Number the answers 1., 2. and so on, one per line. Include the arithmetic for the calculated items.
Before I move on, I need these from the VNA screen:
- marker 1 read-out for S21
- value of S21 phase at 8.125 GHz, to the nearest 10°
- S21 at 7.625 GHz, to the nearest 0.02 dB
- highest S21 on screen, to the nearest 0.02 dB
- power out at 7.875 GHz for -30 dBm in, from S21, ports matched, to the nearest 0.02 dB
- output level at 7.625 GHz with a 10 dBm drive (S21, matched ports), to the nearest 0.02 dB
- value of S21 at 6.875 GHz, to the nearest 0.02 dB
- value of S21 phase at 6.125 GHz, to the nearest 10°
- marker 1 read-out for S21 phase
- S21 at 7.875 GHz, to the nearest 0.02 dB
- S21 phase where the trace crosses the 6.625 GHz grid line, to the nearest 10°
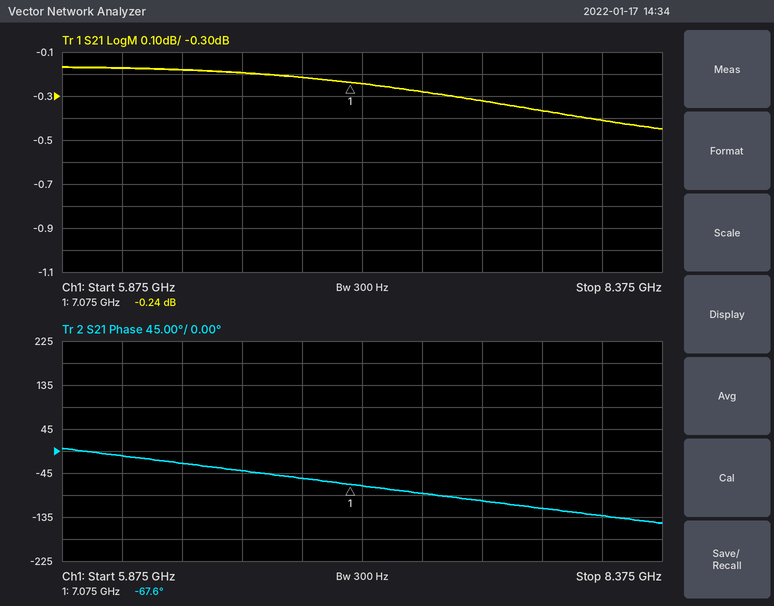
1. -0.24 dB
2. -130°
3. -0.32 dB
4. -0.16 dB
5. -30 dBm + (-0.36 dB) = -30.36 dBm
6. 10 dBm + (-0.32 dB) = 9.68 dBm
7. -0.22 dB
8. -10°
9. -67.6°
10. -0.36 dB
11. -40°
